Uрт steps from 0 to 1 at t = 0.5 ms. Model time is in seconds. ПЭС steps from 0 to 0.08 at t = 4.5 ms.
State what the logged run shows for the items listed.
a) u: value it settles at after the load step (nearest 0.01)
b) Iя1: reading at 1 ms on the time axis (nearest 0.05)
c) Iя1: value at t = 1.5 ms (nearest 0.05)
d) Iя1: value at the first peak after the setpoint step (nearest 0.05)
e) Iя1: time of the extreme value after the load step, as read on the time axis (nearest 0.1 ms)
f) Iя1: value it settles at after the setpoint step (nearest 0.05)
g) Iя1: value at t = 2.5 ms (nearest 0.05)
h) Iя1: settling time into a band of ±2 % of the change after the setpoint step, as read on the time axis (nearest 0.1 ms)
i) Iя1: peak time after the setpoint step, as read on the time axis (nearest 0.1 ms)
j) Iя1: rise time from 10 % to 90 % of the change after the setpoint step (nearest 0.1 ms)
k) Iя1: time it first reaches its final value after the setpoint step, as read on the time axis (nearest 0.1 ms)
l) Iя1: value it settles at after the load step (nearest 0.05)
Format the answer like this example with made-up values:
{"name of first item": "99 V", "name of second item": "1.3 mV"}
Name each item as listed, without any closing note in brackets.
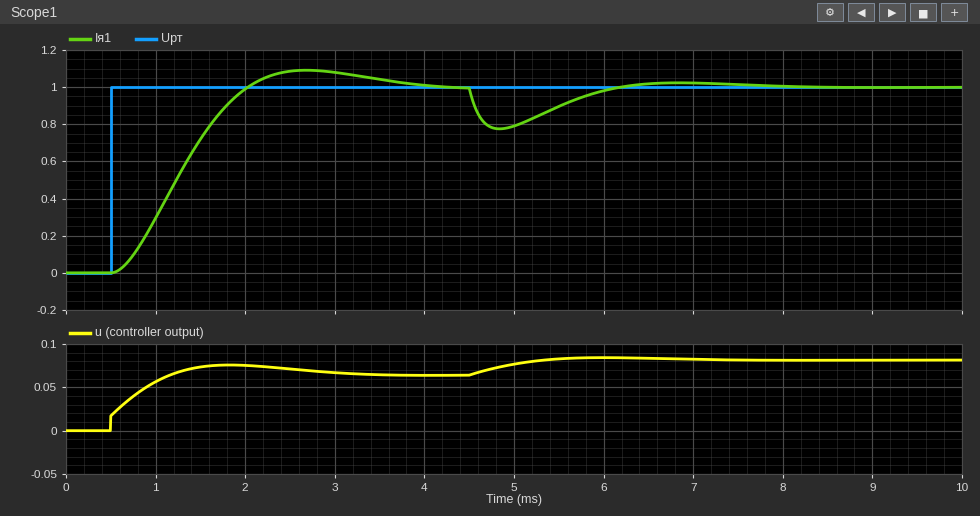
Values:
{"u: value it settles at after the load step": "0.08", "Iя1: reading at 1 ms on the time axis": "0.30", "Iя1: value at t = 1.5 ms": "0.70", "Iя1: value at the first peak after the setpoint step": "1.10", "Iя1: time of the extreme value after the load step, as read on the time axis": "4.8 ms", "Iя1: value it settles at after the setpoint step": "1.00", "Iя1: value at t = 2.5 ms": "1.10", "Iя1: settling time into a band of ±2 % of the change after the setpoint step, as read on the time axis": "3.8 ms", "Iя1: peak time after the setpoint step, as read on the time axis": "2.7 ms", "Iя1: rise time from 10 % to 90 % of the change after the setpoint step": "1.0 ms", "Iя1: time it first reaches its final value after the setpoint step, as read on the time axis": "2.0 ms", "Iя1: value it settles at after the load step": "1.00"}
